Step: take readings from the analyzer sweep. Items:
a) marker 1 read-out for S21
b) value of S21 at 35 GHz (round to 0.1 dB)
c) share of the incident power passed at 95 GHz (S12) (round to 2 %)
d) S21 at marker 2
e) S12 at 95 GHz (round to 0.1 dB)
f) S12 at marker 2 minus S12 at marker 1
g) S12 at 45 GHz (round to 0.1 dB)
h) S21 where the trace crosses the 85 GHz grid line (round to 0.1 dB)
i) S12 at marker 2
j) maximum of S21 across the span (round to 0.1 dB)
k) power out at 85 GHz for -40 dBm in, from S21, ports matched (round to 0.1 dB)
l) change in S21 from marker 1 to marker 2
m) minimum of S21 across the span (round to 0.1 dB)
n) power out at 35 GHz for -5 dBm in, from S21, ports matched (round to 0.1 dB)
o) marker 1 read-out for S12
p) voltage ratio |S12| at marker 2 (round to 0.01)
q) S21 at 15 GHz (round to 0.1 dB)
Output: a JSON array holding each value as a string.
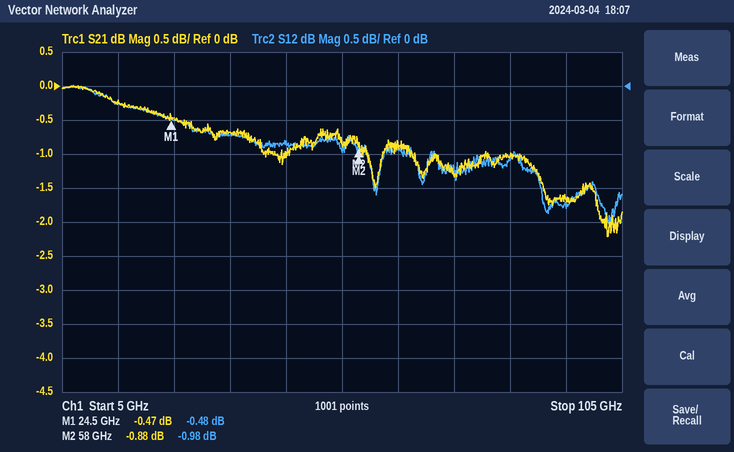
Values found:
["-0.47 dB", "-0.7 dB", "66 %", "-0.88 dB", "-1.8 dB", "-0.50 dB", "-0.8 dB", "-1.0 dB", "-0.98 dB", "0.0 dB", "-41.0 dBm", "-0.41 dB", "-2.2 dB", "-5.7 dBm", "-0.48 dB", "0.89", "-0.2 dB"]
